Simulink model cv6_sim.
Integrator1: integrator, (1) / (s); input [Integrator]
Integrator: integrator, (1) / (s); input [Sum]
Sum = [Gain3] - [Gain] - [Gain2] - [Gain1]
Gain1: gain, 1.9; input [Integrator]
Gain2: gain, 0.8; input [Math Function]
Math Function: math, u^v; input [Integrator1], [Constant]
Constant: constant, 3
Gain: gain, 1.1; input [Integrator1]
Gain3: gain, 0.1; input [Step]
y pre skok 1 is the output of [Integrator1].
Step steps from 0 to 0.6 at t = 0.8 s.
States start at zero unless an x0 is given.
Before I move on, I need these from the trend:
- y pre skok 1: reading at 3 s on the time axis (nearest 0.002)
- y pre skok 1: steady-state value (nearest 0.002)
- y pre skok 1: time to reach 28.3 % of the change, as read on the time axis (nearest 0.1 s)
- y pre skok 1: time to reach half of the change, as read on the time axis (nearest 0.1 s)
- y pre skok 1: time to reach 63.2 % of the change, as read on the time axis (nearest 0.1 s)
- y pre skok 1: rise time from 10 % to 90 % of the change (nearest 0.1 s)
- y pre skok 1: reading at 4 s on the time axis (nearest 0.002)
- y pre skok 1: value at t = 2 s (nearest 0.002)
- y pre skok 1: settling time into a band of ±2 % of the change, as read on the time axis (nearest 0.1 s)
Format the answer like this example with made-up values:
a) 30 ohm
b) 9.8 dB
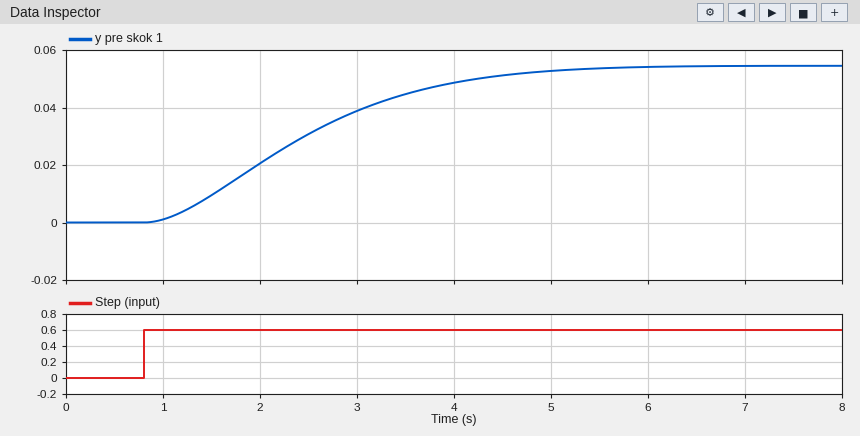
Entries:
a) 0.038
b) 0.054
c) 1.8 s
d) 2.3 s
e) 2.7 s
f) 2.8 s
g) 0.048
h) 0.020
i) 5.3 s
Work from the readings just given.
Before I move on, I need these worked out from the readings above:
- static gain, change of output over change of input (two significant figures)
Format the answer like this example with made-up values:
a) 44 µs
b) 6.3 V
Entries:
a) 0.090
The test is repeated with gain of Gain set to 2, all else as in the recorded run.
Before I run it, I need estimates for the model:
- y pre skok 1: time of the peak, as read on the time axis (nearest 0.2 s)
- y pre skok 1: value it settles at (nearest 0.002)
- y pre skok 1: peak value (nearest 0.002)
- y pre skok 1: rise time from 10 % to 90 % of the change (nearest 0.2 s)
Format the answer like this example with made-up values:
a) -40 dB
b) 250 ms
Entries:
a) 3.8 s
b) 0.030
c) 0.032
d) 1.4 s
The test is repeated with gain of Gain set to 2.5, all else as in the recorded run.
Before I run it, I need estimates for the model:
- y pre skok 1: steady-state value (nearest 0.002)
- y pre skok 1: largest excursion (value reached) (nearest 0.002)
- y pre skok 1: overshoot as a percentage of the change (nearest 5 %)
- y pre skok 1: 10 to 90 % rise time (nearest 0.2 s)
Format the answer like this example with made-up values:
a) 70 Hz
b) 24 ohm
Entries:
a) 0.024
b) 0.026
c) 10 %
d) 1.2 s
